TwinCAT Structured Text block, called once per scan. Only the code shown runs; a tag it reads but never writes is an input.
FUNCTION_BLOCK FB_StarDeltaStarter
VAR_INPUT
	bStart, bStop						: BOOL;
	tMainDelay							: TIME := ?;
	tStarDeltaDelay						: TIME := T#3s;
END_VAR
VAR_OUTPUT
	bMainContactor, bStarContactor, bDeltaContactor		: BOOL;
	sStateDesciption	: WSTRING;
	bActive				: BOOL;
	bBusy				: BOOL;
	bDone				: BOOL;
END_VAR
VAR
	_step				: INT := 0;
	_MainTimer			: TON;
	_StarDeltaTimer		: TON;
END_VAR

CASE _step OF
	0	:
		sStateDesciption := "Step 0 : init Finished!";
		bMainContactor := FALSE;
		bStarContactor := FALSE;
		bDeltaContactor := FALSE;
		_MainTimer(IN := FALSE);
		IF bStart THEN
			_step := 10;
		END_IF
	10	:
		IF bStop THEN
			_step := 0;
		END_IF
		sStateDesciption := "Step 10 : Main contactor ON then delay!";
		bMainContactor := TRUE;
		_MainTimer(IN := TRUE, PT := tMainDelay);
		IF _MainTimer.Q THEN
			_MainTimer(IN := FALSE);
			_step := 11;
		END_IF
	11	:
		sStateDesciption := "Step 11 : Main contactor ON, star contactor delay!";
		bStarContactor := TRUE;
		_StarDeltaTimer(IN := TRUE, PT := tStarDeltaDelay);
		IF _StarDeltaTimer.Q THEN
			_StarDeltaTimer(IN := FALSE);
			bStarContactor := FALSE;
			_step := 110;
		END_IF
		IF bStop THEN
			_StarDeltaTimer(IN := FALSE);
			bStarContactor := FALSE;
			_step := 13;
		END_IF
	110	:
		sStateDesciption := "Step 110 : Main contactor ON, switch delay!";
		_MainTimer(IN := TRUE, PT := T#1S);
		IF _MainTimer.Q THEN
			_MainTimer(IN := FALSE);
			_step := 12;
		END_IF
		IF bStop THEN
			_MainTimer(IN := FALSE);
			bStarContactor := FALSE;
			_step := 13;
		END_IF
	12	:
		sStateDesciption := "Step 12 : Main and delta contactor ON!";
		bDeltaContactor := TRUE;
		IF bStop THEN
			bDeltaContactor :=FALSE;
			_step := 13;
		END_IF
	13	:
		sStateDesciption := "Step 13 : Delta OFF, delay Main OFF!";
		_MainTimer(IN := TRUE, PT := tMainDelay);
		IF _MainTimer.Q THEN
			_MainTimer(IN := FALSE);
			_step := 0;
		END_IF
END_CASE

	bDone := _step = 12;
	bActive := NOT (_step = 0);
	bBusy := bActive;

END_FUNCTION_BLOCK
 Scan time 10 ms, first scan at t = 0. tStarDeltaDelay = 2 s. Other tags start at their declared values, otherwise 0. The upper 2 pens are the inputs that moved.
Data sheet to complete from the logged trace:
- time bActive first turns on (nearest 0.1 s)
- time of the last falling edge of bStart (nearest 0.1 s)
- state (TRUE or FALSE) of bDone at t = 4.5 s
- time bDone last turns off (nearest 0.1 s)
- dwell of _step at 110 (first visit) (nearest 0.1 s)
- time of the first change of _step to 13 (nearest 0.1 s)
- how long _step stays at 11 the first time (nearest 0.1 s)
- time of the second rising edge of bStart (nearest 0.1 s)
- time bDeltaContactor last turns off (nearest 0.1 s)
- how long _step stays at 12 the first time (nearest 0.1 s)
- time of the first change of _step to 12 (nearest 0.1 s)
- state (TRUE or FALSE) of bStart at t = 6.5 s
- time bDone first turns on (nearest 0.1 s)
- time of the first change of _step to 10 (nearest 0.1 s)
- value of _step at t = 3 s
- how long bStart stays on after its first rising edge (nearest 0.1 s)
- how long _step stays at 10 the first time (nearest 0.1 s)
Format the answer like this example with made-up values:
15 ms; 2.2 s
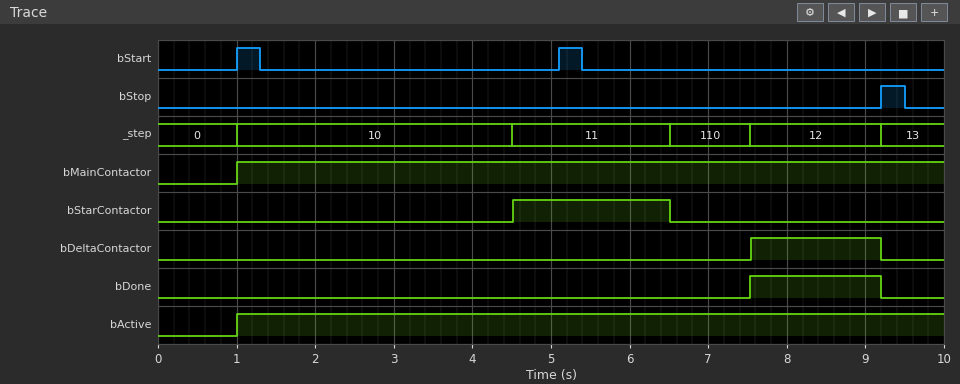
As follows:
1.0 s; 5.4 s; FALSE; 9.2 s; 1.0 s; 9.2 s; 2.0 s; 5.1 s; 9.2 s; 1.7 s; 7.5 s; FALSE; 7.5 s; 1.0 s; 10; 0.3 s; 3.5 s
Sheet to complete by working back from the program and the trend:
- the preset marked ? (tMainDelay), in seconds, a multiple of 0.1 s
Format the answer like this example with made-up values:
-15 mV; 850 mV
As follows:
3.5 s
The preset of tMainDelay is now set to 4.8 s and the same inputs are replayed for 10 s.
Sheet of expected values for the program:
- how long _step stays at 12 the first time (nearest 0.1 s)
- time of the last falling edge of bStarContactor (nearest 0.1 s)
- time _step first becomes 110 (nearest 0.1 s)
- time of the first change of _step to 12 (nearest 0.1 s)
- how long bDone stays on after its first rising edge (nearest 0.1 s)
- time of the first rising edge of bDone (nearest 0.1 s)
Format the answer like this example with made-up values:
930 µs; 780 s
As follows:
0.4 s; 7.8 s; 7.8 s; 8.8 s; 0.4 s; 8.8 s
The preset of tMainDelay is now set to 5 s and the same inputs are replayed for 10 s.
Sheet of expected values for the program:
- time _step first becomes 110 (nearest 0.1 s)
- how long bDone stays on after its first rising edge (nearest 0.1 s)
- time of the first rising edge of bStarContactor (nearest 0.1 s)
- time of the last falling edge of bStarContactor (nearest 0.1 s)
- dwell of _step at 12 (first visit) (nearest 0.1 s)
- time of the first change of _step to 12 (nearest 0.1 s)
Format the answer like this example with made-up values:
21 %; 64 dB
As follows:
8.0 s; 0.2 s; 6.0 s; 8.0 s; 0.2 s; 9.0 s
